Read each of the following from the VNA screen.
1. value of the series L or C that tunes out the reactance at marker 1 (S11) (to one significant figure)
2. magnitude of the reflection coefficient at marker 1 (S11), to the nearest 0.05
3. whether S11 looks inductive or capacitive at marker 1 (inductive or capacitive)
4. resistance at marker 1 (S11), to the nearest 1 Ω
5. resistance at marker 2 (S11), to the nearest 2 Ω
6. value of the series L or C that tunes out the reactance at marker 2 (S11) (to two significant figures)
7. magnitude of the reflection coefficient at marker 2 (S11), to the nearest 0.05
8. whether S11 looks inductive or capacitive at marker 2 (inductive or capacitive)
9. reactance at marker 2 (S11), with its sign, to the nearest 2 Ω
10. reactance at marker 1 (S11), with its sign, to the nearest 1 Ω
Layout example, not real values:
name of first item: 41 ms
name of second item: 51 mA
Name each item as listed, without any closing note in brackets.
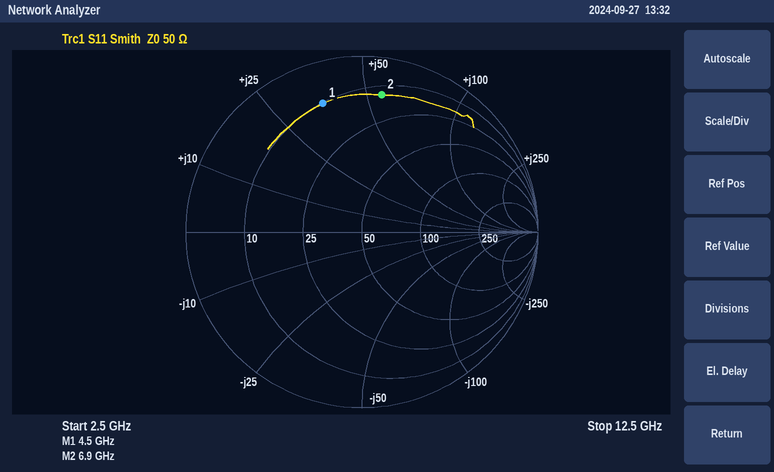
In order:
value of the series L or C that tunes out the reactance at marker 1 (S11): 1.0 pF
magnitude of the reflection coefficient at marker 1 (S11), to the nearest 0.05: 0.75
whether S11 looks inductive or capacitive at marker 1: inductive
resistance at marker 1 (S11), to the nearest 1 Ω: 10 Ω
resistance at marker 2 (S11), to the nearest 2 Ω: 14 Ω
value of the series L or C that tunes out the reactance at marker 2 (S11): 410 fF
magnitude of the reflection coefficient at marker 2 (S11), to the nearest 0.05: 0.80
whether S11 looks inductive or capacitive at marker 2: inductive
reactance at marker 2 (S11), with its sign, to the nearest 2 Ω: +56 Ω
reactance at marker 1 (S11), with its sign, to the nearest 1 Ω: +36 Ω
